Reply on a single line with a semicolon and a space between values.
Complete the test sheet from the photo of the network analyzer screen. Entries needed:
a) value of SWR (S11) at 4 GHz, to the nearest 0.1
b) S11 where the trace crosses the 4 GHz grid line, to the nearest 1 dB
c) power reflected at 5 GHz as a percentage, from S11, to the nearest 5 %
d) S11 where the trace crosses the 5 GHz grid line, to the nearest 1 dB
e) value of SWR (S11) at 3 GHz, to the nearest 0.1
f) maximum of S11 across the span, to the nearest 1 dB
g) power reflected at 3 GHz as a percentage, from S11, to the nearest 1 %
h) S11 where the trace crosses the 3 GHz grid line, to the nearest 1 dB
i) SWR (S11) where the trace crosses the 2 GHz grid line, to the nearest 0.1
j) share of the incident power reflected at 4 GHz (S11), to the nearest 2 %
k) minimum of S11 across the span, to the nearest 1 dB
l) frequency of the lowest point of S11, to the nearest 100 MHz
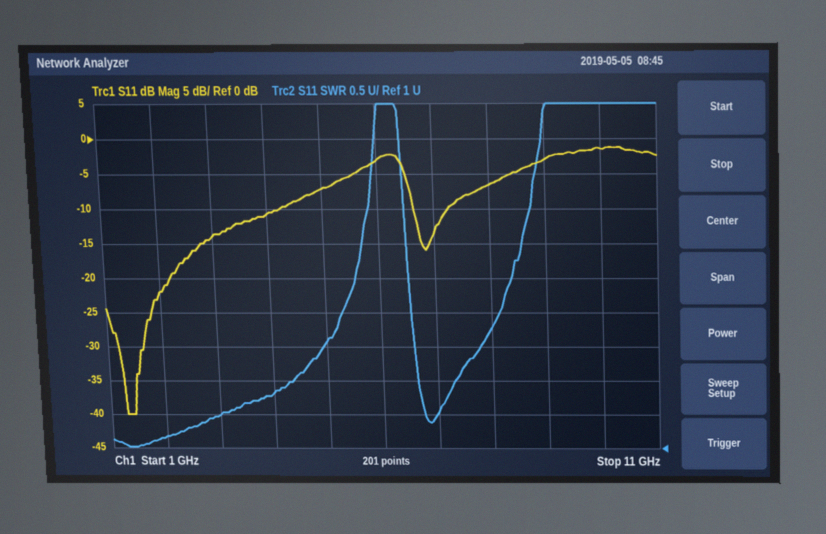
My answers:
1.8; -11 dB; 20 %; -7 dB; 1.5; -1 dB; 4 %; -14 dB; 1.2; 8 %; -40 dB; 1.3 GHz
